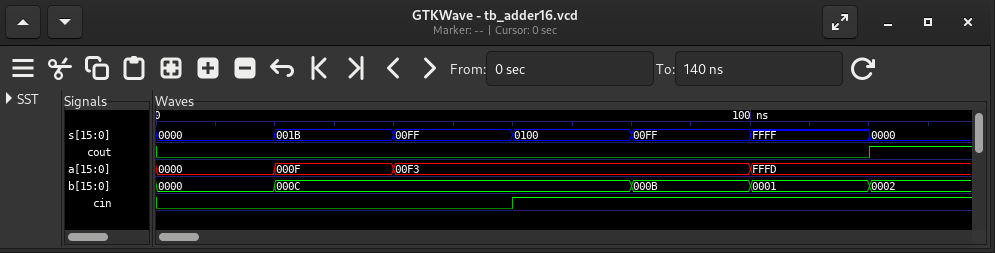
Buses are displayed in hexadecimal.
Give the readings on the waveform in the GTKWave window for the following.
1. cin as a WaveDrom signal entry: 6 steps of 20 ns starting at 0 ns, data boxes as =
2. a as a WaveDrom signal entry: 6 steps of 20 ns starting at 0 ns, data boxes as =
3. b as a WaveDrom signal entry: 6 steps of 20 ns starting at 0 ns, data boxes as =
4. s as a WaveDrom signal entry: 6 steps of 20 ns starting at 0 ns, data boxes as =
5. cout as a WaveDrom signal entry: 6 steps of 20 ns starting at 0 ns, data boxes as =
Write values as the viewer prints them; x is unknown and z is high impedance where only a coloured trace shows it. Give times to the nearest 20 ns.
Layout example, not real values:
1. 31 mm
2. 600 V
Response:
1. {name: 'cin', wave: '0..1..'}
2. {name: 'a', wave: '===..=', data: '0000 000F 00F3 FFFD'}
3. {name: 'b', wave: '==..==', data: '0000 000C 000B 0001'}
4. {name: 's', wave: '======', data: '0000 001B 00FF 0100 00FF FFFF'}
5. {name: 'cout', wave: '0.....'}
